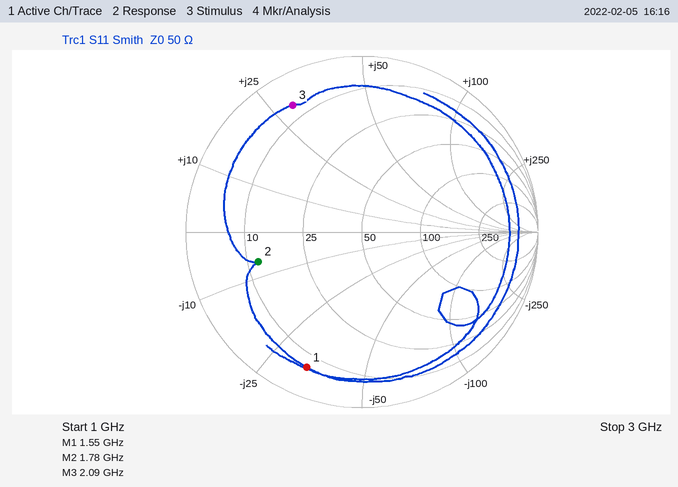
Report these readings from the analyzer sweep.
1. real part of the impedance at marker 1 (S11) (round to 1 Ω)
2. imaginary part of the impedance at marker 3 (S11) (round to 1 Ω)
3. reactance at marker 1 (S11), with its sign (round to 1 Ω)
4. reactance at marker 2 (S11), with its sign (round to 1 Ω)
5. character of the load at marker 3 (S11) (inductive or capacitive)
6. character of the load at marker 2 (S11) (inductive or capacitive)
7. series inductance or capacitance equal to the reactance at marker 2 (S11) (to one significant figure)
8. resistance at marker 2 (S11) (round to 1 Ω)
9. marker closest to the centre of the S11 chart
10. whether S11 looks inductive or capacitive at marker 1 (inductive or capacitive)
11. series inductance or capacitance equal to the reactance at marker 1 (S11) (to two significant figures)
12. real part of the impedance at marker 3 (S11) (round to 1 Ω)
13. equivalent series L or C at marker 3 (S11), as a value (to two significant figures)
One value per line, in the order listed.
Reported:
7 Ω
+29 Ω
-33 Ω
-7 Ω
inductive
capacitive
10 pF
12 Ω
marker 2
capacitive
3.1 pF
7 Ω
2.2 nH
